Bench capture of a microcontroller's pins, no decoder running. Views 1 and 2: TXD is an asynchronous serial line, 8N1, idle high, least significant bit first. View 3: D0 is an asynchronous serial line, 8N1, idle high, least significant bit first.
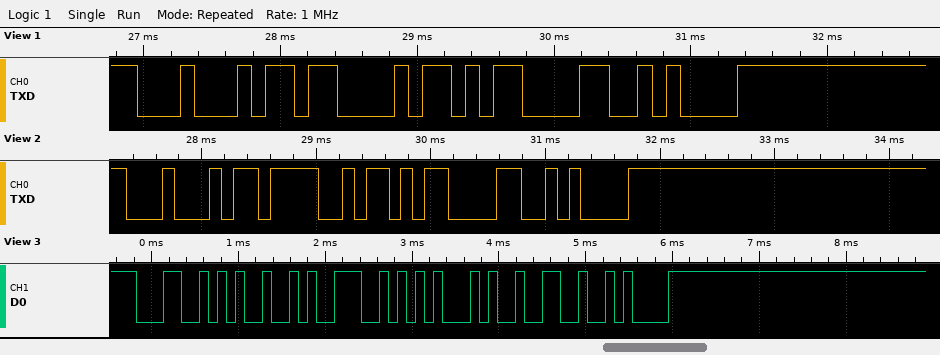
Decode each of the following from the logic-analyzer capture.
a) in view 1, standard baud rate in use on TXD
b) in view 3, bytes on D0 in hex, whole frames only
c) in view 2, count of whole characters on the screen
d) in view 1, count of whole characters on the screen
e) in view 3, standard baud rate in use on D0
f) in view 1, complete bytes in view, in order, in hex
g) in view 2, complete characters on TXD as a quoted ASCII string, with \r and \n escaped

9600 baud
4C 49 4E 45 32 0A
4
4
9600 baud
44 43 0D 0A
"DO\r\n"
